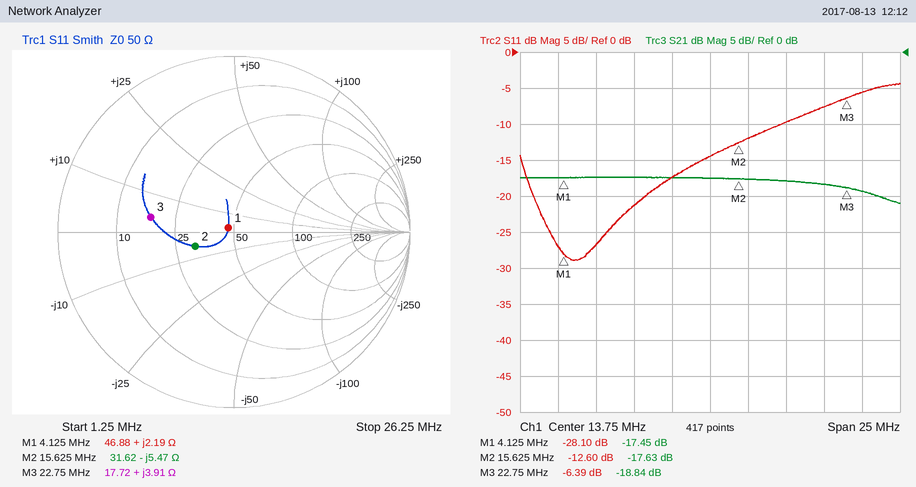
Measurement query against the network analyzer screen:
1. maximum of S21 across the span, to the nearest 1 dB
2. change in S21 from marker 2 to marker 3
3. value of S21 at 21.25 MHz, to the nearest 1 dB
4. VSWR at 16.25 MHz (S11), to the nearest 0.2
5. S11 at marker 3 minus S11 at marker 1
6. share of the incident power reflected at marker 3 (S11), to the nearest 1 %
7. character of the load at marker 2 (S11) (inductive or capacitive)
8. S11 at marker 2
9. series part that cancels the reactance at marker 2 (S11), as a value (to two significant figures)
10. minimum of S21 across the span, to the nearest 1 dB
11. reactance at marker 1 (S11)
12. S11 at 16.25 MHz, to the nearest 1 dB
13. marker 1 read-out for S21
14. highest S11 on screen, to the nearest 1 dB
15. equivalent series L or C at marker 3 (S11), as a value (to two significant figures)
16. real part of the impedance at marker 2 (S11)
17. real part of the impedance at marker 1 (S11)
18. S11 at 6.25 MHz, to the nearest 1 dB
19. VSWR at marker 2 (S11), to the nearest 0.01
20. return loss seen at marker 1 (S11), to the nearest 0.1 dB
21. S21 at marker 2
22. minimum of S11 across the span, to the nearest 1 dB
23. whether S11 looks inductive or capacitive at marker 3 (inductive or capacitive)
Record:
-17 dB
-1.21 dB
-18 dB
1.6
21.71 dB
23 %
capacitive
-12.60 dB
56 nH
-21 dB
+2.19 Ω
-12 dB
-17.45 dB
-4 dB
27 nH
31.62 Ω
46.88 Ω
-27 dB
1.61
28.1 dB
-17.63 dB
-29 dB
inductive
